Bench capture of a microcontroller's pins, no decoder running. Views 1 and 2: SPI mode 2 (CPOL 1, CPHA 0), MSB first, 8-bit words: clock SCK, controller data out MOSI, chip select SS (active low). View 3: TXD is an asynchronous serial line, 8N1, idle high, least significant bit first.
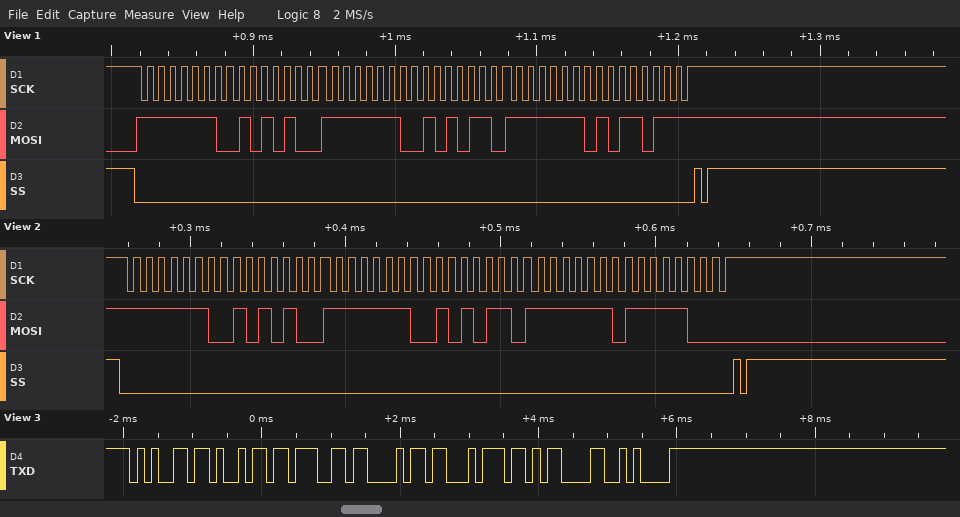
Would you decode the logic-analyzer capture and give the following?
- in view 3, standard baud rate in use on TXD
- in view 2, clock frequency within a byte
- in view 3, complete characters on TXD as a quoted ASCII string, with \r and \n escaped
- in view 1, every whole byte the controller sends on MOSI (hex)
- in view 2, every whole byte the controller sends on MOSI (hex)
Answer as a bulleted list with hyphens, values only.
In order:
- 9600 baud
- 125 kHz
- "eight\r\n"
- FE 54 FE 56 FE B7
- 0xFE 0x54 0xFE 0x56 0xFE 0xF8
